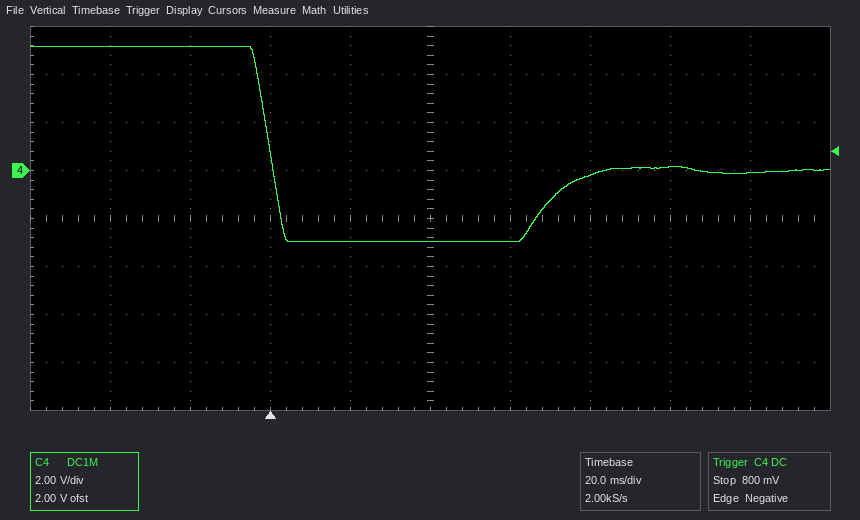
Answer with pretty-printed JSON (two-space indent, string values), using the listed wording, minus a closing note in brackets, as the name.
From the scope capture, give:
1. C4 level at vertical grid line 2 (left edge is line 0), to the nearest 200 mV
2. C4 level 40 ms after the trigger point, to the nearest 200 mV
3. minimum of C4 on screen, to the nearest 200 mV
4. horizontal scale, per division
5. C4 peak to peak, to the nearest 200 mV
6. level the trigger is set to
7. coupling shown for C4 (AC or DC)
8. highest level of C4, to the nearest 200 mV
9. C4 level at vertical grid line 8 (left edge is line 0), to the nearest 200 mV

{
  "C4 level at vertical grid line 2 (left edge is line 0), to the nearest 200 mV": "5.2 V",
  "C4 level 40 ms after the trigger point, to the nearest 200 mV": "-3.0 V",
  "minimum of C4 on screen, to the nearest 200 mV": "-3.0 V",
  "horizontal scale, per division": "20 ms",
  "C4 peak to peak, to the nearest 200 mV": "8.2 V",
  "level the trigger is set to": "800 mV",
  "coupling shown for C4": "DC",
  "highest level of C4, to the nearest 200 mV": "5.2 V",
  "C4 level at vertical grid line 8 (left edge is line 0), to the nearest 200 mV": "200 mV"
}
